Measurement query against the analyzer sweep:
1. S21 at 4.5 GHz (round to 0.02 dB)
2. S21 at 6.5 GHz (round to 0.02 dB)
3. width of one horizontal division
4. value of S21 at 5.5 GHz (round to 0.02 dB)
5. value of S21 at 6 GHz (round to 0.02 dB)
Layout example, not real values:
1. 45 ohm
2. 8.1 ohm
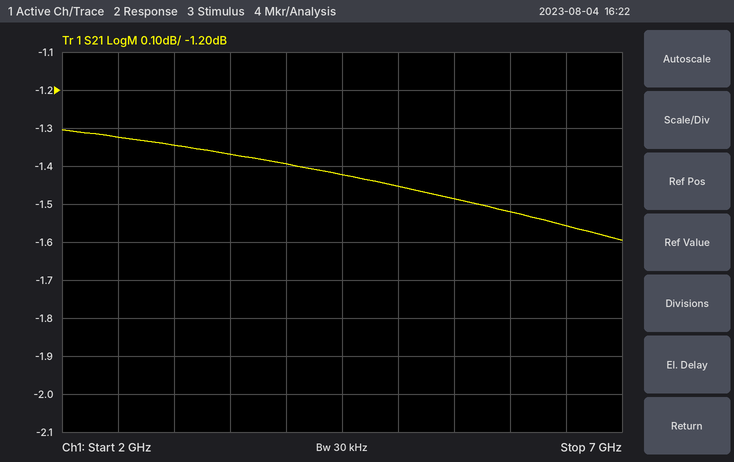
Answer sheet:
1. -1.42 dB
2. -1.56 dB
3. 500 MHz
4. -1.48 dB
5. -1.52 dB
